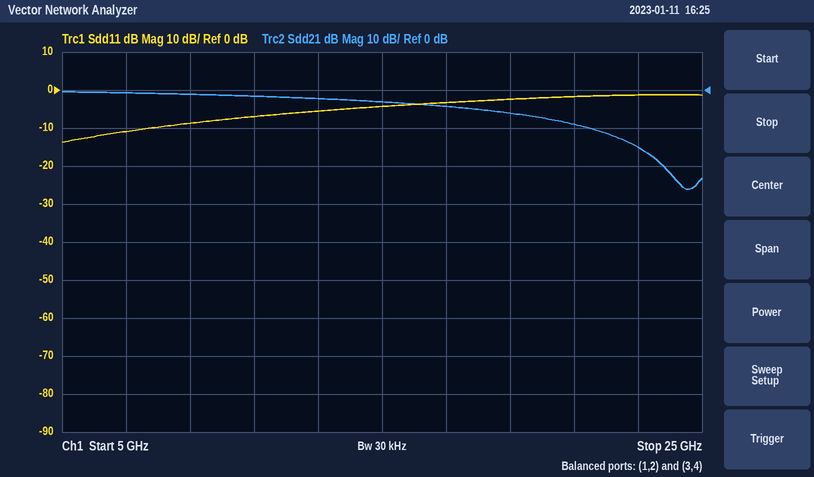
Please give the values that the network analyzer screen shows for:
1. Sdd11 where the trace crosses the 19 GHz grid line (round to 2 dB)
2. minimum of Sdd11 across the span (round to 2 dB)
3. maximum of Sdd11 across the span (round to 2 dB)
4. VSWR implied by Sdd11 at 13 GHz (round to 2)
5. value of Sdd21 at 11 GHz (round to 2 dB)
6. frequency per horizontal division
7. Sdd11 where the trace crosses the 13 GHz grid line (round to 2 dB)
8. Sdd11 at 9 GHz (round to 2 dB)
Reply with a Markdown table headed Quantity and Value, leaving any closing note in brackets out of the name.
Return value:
| Quantity | Value |
|---|---|
| Sdd11 where the trace crosses the 19 GHz grid line | -2 dB |
| minimum of Sdd11 across the span | -14 dB |
| maximum of Sdd11 across the span | -2 dB |
| VSWR implied by Sdd11 at 13 GHz | 4 |
| value of Sdd21 at 11 GHz | -2 dB |
| frequency per horizontal division | 2 GHz |
| Sdd11 where the trace crosses the 13 GHz grid line | -6 dB |
| Sdd11 at 9 GHz | -8 dB |
